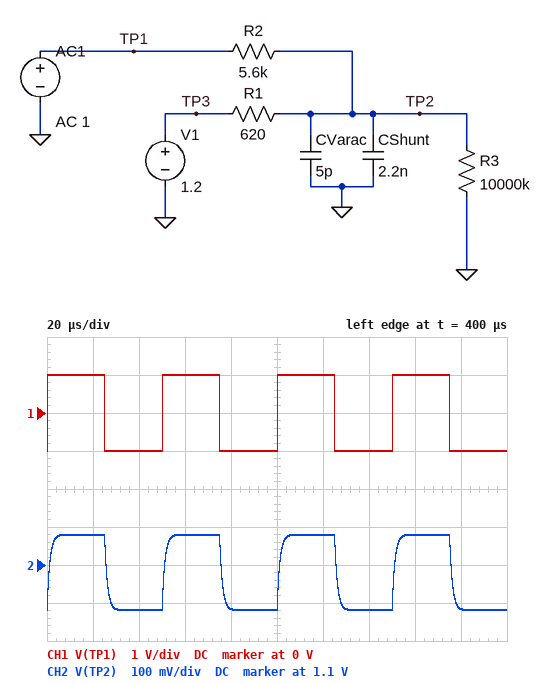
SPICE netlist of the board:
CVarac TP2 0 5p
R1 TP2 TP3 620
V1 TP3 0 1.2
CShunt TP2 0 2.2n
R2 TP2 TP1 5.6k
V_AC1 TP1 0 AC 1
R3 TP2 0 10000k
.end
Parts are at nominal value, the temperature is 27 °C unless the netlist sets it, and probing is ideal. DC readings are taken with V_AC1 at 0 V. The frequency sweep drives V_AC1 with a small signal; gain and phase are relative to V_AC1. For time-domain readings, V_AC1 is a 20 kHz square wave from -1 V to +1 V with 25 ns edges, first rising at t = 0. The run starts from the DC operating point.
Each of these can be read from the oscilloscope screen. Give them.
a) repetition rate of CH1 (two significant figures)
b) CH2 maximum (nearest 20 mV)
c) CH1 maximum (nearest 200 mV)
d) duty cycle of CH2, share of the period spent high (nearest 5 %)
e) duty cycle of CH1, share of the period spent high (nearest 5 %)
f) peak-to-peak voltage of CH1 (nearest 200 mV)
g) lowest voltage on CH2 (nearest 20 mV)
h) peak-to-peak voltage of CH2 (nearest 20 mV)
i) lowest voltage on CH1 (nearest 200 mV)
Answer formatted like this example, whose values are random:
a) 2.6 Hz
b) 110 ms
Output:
a) 20 kHz
b) 1.18 V
c) 1.0 V
d) 50 %
e) 50 %
f) 2.0 V
g) 980 mV
h) 200 mV
i) -1.0 V
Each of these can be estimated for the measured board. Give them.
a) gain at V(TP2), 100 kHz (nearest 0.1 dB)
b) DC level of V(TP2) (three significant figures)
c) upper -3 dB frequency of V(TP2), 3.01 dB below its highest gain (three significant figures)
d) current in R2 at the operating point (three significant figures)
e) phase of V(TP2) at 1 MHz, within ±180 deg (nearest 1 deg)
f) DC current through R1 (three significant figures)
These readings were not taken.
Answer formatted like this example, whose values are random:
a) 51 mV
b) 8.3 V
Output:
a) -22.1 dB
b) 1.08 V
c) 129 kHz
d) 193 µA
e) -83 deg
f) 193 µA
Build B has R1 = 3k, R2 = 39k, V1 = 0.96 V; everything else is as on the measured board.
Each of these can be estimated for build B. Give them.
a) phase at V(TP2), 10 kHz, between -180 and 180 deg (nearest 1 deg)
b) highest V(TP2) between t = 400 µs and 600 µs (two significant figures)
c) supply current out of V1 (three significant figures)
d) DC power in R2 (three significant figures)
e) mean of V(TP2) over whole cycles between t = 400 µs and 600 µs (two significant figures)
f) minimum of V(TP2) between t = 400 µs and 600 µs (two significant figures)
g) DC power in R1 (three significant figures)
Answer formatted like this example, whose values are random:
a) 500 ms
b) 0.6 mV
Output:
a) -21 deg
b) 960 mV
c) 22.9 µA
d) 20.4 µW
e) 890 mV
f) 820 mV
g) 1.58 µW
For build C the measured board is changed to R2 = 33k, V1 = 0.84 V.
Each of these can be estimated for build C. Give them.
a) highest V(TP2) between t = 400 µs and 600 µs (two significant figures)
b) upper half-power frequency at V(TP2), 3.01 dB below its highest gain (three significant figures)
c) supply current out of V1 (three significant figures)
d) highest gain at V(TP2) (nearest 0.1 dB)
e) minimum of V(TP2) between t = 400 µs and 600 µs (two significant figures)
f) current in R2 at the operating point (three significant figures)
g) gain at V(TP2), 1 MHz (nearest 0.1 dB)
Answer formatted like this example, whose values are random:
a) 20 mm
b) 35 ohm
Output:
a) 840 mV
b) 119 kHz
c) 25.1 µA
d) -34.7 dB
e) 810 mV
f) 25.0 µA
g) -53.3 dB
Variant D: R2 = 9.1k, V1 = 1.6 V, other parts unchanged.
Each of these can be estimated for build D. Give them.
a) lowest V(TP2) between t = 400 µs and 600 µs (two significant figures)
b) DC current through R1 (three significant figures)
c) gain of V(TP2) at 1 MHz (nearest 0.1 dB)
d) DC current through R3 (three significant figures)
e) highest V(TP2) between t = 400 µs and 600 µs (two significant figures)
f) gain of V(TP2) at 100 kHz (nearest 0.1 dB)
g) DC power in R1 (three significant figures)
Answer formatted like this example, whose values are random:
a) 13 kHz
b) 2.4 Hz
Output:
a) 1.4 V
b) 165 µA
c) -42.1 dB
d) 150 nA
e) 1.6 V
f) -26.1 dB
g) 16.8 µW
